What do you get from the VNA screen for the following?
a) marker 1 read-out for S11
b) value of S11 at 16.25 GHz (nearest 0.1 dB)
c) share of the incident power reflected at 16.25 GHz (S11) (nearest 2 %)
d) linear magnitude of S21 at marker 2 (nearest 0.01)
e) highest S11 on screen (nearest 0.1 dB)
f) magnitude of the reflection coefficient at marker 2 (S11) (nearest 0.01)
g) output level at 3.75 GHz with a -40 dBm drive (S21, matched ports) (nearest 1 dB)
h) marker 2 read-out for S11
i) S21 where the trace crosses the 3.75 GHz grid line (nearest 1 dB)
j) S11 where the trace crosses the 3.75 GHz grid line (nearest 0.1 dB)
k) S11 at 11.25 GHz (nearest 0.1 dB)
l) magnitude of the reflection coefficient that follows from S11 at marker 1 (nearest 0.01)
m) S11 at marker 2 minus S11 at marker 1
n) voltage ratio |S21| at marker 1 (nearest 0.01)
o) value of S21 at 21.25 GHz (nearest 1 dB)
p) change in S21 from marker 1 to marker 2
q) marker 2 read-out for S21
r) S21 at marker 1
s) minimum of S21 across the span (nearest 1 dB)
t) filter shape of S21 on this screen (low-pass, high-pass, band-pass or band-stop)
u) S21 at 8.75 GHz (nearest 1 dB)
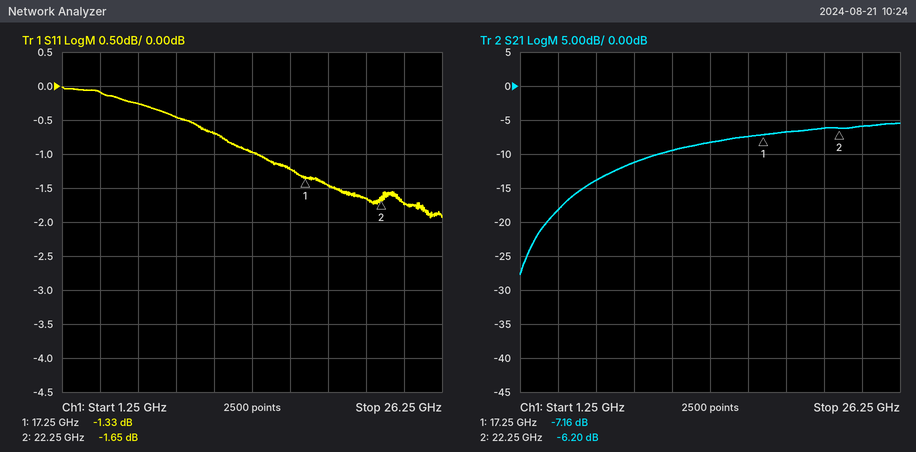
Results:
-1.33 dB
-1.2 dB
76 %
0.49
0.0 dB
0.83
-58 dBm
-1.65 dB
-18 dB
-0.1 dB
-0.7 dB
0.86
-0.32 dB
0.44
-6 dB
0.96 dB
-6.20 dB
-7.16 dB
-28 dB
high-pass
-11 dB
